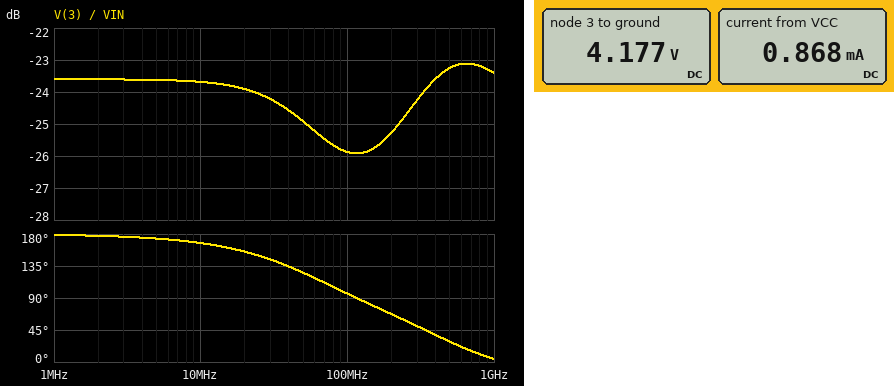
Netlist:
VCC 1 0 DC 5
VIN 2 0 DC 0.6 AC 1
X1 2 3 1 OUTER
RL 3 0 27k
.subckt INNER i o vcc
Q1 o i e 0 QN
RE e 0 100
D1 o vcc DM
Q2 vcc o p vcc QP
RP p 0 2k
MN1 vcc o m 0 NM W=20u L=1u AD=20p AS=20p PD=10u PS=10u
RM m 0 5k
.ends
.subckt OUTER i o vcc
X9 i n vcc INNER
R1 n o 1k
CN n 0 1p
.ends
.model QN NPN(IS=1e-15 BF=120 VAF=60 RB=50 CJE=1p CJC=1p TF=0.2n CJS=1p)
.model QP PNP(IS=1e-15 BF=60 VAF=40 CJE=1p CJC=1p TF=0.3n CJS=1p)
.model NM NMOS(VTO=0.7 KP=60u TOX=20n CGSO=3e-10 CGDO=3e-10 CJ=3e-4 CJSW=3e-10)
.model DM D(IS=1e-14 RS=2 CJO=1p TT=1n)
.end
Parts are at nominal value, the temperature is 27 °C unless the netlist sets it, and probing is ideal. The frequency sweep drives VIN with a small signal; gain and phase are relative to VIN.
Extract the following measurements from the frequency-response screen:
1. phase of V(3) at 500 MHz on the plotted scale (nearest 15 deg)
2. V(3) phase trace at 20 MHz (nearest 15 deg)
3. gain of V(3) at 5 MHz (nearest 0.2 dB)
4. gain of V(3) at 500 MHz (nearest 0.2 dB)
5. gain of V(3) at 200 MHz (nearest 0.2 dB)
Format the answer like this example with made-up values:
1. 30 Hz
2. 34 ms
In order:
1. 30 deg
2. 150 deg
3. -23.6 dB
4. -23.2 dB
5. -25.2 dB
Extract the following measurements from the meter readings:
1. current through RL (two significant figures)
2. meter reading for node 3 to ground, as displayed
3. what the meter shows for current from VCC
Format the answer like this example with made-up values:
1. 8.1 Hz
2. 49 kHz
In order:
1. 150 µA
2. 4.177 V
3. 0.868 mA
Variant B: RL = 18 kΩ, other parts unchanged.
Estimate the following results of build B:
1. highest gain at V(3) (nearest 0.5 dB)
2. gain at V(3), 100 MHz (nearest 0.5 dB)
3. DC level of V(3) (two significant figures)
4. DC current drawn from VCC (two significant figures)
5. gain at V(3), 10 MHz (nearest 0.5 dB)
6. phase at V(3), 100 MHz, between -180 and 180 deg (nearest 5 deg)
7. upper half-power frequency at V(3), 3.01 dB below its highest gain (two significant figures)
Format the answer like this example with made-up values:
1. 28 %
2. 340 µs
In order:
1. -24.0 dB
2. -28.5 dB
3. 4.1 V
4. 1.0 mA
5. -27.0 dB
6. 100 deg
7. 8.0 GHz
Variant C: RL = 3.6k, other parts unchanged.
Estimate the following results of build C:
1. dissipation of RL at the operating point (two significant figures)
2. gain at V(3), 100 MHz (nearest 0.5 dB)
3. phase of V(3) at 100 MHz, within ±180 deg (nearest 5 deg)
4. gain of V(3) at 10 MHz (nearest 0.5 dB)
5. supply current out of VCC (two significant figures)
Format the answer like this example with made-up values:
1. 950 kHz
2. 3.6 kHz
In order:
1. 3.1 mW
2. -41.5 dB
3. 110 deg
4. -40.5 dB
5. 2.4 mA
